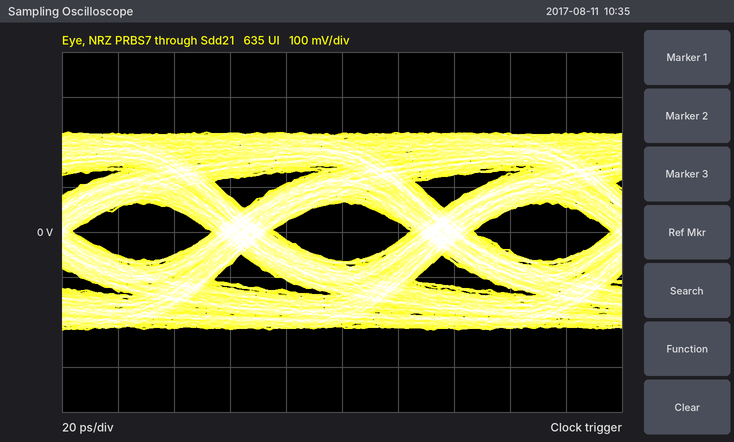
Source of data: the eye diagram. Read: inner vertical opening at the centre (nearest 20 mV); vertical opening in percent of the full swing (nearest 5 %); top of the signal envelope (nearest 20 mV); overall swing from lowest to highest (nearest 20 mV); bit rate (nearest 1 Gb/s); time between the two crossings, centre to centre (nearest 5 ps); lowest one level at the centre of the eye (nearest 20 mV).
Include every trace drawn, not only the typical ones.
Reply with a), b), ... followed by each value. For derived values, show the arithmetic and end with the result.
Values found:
a) 140 mV
b) 140 mV / 440 mV ≈ 31.8 %, so 30 % to the nearest 5 %
c) 220 mV
d) 440 mV
e) 14 Gb/s
f) 70 ps
g) 60 mV
